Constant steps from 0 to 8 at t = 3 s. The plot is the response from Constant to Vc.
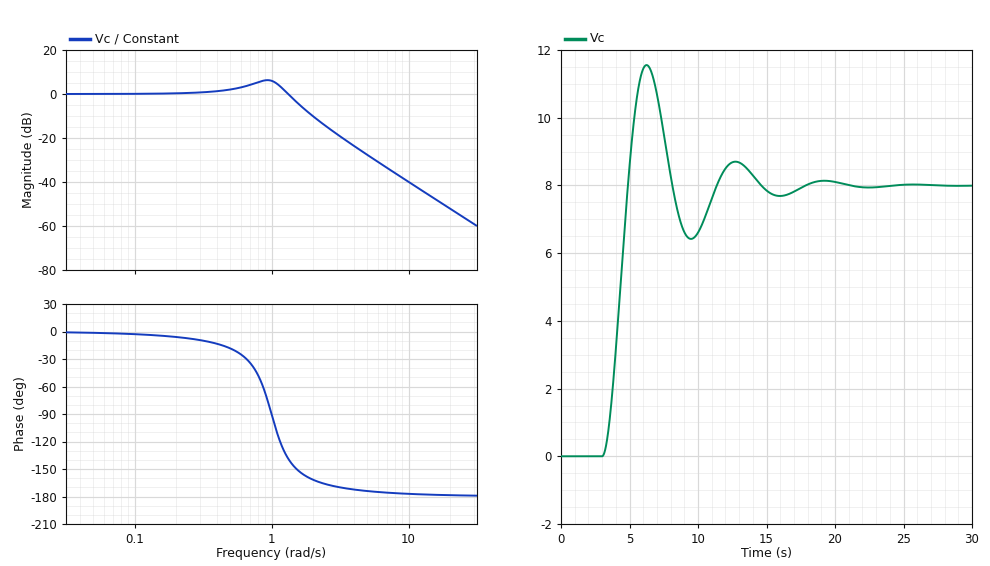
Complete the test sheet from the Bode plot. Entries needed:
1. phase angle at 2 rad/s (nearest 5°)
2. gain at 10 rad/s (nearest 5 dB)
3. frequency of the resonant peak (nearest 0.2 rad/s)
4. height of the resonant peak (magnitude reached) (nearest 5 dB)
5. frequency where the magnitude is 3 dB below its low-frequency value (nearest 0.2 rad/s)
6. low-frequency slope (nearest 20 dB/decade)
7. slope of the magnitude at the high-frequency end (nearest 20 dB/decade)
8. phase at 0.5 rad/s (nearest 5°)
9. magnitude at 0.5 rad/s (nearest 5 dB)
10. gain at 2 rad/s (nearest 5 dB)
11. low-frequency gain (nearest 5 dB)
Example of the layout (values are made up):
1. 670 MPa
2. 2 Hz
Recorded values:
1. -160°
2. -40 dB
3. 1.0 rad/s
4. 5 dB
5. 1.4 rad/s
6. 0 dB/decade
7. -40 dB/decade
8. -20°
9. 0 dB
10. -10 dB
11. 0 dB
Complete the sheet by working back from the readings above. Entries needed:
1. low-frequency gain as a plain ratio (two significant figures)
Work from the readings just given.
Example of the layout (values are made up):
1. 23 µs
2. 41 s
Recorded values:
1. 1.0
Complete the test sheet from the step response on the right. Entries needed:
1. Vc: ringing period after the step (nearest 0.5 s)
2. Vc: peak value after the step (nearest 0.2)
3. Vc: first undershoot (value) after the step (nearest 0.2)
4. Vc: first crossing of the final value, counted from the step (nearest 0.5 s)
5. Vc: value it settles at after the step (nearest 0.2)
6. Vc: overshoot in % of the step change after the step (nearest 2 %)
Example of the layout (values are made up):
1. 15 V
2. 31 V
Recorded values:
1. 6.5 s
2. 11.6
3. 6.4
4. 2.0 s
5. 8.0
6. 44 %
